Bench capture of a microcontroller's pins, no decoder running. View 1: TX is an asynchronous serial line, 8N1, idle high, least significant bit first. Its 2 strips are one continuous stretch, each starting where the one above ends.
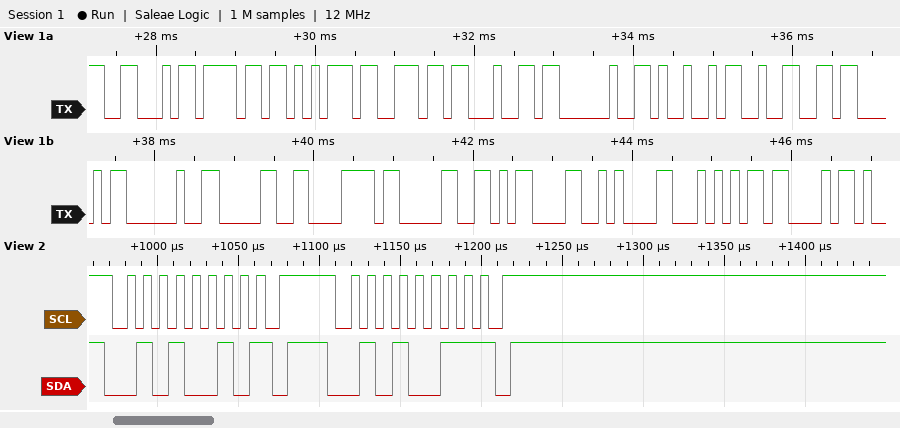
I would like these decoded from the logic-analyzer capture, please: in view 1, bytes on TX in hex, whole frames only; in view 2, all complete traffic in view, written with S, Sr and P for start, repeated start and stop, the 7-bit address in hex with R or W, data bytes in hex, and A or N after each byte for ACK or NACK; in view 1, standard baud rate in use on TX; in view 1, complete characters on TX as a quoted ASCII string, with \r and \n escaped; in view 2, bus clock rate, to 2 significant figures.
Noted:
46 6F 75 6E 64 20 49 32 43 20 30 78 30 0D 0A 54 43
S 29W N P S 29R N P
9600 baud
"Found I2C 0x0\r\nTC"
100 kHz
